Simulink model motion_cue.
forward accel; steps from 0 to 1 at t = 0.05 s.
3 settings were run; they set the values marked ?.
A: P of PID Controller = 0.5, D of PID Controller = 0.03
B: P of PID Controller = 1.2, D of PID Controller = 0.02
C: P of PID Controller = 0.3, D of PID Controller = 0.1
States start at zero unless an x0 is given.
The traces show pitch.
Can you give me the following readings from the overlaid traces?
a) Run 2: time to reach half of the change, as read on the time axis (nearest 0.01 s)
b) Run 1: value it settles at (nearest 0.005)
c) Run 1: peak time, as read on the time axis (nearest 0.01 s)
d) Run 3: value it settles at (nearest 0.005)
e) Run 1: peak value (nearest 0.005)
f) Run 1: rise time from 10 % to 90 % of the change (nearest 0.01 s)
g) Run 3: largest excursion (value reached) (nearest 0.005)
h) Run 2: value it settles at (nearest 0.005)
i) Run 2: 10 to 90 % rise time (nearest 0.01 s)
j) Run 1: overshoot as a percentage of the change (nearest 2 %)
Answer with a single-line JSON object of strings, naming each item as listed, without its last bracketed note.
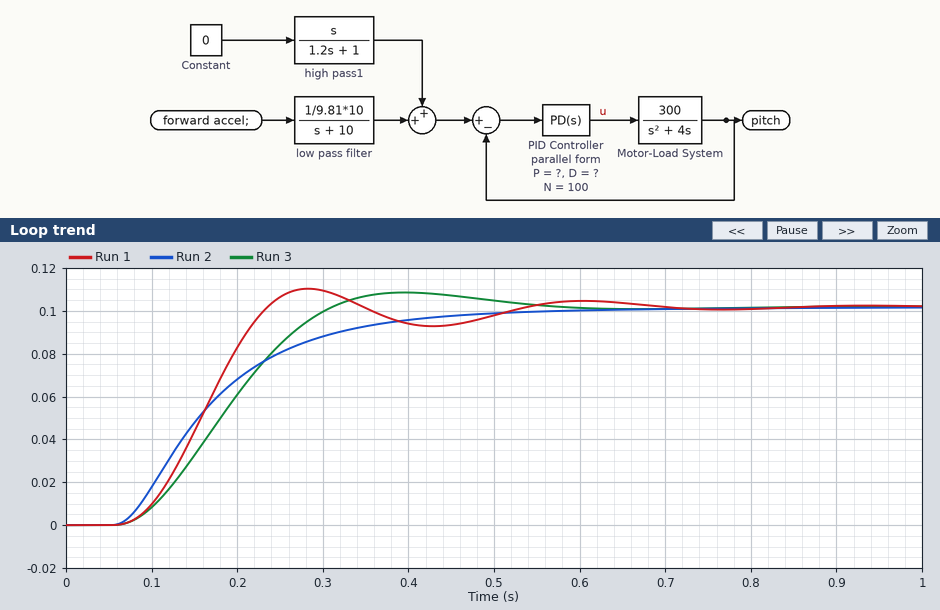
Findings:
{"Run 2: time to reach half of the change, as read on the time axis": "0.16 s", "Run 1: value it settles at": "0.100", "Run 1: peak time, as read on the time axis": "0.28 s", "Run 3: value it settles at": "0.100", "Run 1: peak value": "0.110", "Run 1: rise time from 10 % to 90 % of the change": "0.11 s", "Run 3: largest excursion (value reached)": "0.110", "Run 2: value it settles at": "0.100", "Run 2: 10 to 90 % rise time": "0.25 s", "Run 1: overshoot as a percentage of the change": "8 %"}
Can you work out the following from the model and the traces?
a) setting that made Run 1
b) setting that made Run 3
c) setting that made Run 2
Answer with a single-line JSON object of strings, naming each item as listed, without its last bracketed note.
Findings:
{"setting that made Run 1": "B", "setting that made Run 3": "A", "setting that made Run 2": "C"}
